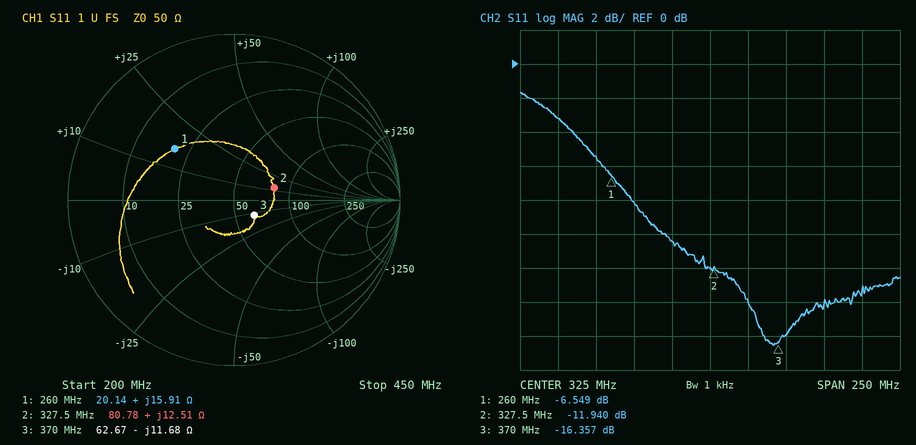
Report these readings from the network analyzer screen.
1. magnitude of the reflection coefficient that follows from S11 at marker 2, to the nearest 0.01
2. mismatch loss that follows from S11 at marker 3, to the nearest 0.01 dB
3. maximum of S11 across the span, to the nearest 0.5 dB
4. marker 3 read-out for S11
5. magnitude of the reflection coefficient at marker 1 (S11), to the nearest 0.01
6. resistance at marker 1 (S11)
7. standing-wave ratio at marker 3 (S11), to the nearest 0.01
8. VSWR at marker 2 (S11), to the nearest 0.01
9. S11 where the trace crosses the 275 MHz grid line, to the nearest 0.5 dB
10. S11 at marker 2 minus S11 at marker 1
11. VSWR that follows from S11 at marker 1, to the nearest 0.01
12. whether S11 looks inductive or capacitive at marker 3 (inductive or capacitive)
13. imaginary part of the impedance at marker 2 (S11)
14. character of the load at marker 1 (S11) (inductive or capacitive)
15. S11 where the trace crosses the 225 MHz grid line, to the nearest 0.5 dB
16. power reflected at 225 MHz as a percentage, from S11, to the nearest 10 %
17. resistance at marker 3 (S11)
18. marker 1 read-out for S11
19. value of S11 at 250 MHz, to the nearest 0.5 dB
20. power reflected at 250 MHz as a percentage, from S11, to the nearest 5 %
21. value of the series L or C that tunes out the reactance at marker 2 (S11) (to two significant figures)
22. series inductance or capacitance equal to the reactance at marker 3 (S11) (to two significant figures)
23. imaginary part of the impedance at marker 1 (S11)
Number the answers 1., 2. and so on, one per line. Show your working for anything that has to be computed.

1. 10^(-11.94/20) ≈ 0.25
2. −10 log10(1 − 10^(-16.357/10)) ≈ 0.10 dB
3. -1.5 dB
4. -16.357 dB
5. 0.47
6. 20.14 Ω
7. 1.36
8. 1.68
9. -8.0 dB
10. -11.94 − (-6.549) = -5.391 dB
11. (1 + 0.4705)/(1 − 0.4705) ≈ 2.78
12. capacitive
13. +12.51 Ω
14. inductive
15. -3.0 dB
16. 10^(-3/10) ≈ 50 %
17. 62.67 Ω
18. -6.549 dB
19. -5.5 dB
20. 10^(-5.5/10) ≈ 28.2 %, so 30 % to the nearest 5 %
21. C = 1/(2π × 327.5 MHz × 12.51 Ω) ≈ 39 pF
22. C = 1/(2π × 370 MHz × 11.68 Ω) ≈ 37 pF
23. +15.91 Ω
